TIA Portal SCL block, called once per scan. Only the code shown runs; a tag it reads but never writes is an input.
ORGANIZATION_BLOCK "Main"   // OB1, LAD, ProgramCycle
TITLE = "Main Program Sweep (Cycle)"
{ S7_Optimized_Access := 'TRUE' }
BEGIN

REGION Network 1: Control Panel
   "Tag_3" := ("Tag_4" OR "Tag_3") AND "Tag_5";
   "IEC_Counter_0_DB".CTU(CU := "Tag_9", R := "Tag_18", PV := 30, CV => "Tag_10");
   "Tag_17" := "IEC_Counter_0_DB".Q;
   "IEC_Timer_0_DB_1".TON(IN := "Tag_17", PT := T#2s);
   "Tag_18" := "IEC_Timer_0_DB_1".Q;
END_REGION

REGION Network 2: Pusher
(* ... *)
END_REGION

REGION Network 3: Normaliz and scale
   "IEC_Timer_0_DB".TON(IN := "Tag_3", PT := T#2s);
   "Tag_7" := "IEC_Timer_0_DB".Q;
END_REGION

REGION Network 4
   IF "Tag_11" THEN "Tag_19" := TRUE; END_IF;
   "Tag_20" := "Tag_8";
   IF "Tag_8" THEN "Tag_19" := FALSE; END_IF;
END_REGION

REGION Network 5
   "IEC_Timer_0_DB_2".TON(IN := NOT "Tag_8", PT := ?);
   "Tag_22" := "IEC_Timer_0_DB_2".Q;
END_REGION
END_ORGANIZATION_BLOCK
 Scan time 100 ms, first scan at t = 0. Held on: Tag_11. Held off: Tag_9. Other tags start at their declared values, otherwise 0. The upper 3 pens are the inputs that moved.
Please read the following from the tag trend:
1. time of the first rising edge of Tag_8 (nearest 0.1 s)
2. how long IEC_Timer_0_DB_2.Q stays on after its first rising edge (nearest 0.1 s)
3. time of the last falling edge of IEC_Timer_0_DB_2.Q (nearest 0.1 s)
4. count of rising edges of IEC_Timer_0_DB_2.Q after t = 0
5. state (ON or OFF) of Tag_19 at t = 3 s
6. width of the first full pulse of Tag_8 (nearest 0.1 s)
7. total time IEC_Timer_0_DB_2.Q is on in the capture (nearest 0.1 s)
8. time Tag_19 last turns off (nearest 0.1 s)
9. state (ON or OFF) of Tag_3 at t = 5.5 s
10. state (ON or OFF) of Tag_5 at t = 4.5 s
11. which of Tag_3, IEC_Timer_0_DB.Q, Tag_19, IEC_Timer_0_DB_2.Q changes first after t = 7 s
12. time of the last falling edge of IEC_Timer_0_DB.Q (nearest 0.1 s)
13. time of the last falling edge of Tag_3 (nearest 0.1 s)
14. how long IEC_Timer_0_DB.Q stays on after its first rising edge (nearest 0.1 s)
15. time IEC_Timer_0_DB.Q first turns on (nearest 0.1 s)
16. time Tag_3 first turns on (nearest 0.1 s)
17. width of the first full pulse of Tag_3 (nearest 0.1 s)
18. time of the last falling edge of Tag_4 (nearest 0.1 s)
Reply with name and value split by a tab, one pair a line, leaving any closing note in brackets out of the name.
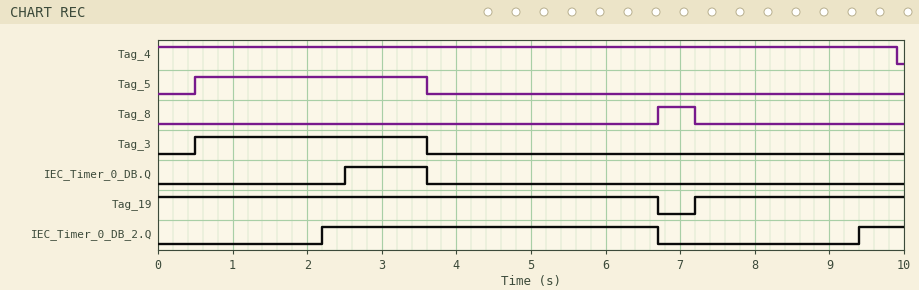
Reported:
time of the first rising edge of Tag_8	6.7 s
how long IEC_Timer_0_DB_2.Q stays on after its first rising edge	4.5 s
time of the last falling edge of IEC_Timer_0_DB_2.Q	6.7 s
count of rising edges of IEC_Timer_0_DB_2.Q after t = 0	2
state (ON or OFF) of Tag_19 at t = 3 s	ON
width of the first full pulse of Tag_8	0.5 s
total time IEC_Timer_0_DB_2.Q is on in the capture	5.1 s
time Tag_19 last turns off	6.7 s
state (ON or OFF) of Tag_3 at t = 5.5 s	OFF
state (ON or OFF) of Tag_5 at t = 4.5 s	OFF
which of Tag_3, IEC_Timer_0_DB.Q, Tag_19, IEC_Timer_0_DB_2.Q changes first after t = 7 s	Tag_19
time of the last falling edge of IEC_Timer_0_DB.Q	3.6 s
time of the last falling edge of Tag_3	3.6 s
how long IEC_Timer_0_DB.Q stays on after its first rising edge	1.1 s
time IEC_Timer_0_DB.Q first turns on	2.5 s
time Tag_3 first turns on	0.5 s
width of the first full pulse of Tag_3	3.1 s
time of the last falling edge of Tag_4	9.9 s
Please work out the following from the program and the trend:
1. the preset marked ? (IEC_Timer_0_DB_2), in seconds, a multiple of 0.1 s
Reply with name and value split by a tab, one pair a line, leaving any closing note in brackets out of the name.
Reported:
the preset marked ? (IEC_Timer_0_DB_2), in seconds, a multiple of 0.1 s	2.2 s
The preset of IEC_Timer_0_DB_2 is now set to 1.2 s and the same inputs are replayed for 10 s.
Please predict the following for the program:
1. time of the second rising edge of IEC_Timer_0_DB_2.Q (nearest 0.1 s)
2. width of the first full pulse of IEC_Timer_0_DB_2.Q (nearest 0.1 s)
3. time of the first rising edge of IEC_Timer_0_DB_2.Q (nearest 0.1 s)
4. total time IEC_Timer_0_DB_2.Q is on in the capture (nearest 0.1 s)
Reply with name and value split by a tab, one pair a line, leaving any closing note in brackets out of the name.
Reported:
time of the second rising edge of IEC_Timer_0_DB_2.Q	8.4 s
width of the first full pulse of IEC_Timer_0_DB_2.Q	5.5 s
time of the first rising edge of IEC_Timer_0_DB_2.Q	1.2 s
total time IEC_Timer_0_DB_2.Q is on in the capture	7.1 s
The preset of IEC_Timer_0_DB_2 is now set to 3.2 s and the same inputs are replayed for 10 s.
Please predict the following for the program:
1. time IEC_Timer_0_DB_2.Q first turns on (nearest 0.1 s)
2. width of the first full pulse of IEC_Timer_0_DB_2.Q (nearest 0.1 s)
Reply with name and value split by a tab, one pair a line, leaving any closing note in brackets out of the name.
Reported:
time IEC_Timer_0_DB_2.Q first turns on	3.2 s
width of the first full pulse of IEC_Timer_0_DB_2.Q	3.5 s
